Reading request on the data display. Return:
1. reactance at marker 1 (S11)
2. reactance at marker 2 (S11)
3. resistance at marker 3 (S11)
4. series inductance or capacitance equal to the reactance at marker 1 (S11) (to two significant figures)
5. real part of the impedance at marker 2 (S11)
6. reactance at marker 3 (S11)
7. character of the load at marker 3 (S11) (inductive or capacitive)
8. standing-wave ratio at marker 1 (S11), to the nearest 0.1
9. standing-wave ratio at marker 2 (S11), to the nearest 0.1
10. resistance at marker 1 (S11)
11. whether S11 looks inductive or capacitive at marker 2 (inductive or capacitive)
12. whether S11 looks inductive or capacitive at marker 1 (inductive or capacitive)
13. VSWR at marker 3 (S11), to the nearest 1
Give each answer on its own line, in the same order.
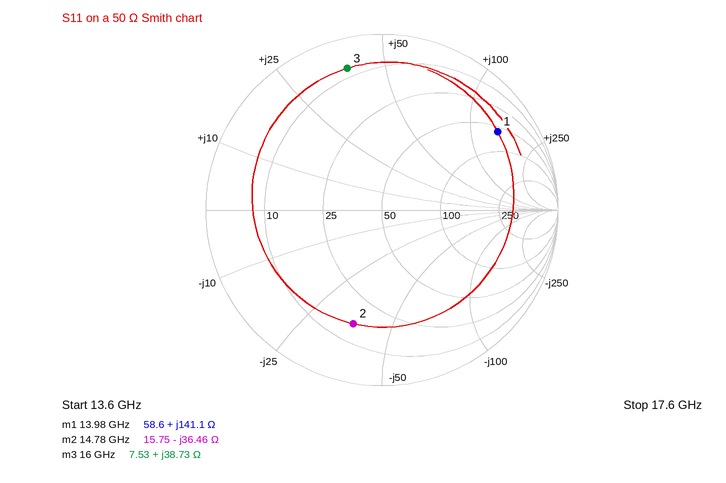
+141.1 Ω
-36.46 Ω
7.53 Ω
1.6 nH
15.75 Ω
+38.73 Ω
inductive
8.7
5.0
58.6 Ω
capacitive
inductive
11
